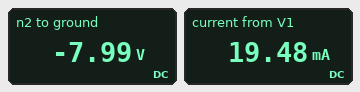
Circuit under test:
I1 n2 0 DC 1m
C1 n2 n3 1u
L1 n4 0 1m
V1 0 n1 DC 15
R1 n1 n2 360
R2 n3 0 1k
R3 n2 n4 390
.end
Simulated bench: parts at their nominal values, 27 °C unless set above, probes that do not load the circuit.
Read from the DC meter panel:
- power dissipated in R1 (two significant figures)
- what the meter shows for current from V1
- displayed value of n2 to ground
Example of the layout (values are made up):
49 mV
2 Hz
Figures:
140 mW
19.48 mA
-7.99 V
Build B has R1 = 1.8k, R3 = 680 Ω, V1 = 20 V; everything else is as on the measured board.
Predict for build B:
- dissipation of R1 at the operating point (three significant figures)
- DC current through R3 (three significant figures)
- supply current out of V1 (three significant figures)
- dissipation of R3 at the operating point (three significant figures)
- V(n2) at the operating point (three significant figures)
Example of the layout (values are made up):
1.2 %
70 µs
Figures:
109 mW
8.79 mA
7.79 mA
52.5 mW
-5.98 V
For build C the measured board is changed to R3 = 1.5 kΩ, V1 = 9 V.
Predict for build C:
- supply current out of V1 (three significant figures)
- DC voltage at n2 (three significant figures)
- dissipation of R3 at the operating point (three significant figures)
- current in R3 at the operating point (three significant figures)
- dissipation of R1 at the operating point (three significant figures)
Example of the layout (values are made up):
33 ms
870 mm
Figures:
4.03 mA
-7.55 V
38.0 mW
5.03 mA
5.85 mW
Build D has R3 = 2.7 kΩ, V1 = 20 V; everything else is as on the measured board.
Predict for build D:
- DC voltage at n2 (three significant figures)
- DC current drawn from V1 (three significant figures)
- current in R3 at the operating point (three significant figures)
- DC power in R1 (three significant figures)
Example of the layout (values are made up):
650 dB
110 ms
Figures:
-18.0 V
5.65 mA
6.65 mA
11.5 mW
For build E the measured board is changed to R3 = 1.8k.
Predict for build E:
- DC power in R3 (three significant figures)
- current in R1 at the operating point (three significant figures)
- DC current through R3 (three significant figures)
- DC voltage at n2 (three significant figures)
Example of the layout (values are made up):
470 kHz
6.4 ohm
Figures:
91.0 mW
6.11 mA
7.11 mA
-12.8 V
